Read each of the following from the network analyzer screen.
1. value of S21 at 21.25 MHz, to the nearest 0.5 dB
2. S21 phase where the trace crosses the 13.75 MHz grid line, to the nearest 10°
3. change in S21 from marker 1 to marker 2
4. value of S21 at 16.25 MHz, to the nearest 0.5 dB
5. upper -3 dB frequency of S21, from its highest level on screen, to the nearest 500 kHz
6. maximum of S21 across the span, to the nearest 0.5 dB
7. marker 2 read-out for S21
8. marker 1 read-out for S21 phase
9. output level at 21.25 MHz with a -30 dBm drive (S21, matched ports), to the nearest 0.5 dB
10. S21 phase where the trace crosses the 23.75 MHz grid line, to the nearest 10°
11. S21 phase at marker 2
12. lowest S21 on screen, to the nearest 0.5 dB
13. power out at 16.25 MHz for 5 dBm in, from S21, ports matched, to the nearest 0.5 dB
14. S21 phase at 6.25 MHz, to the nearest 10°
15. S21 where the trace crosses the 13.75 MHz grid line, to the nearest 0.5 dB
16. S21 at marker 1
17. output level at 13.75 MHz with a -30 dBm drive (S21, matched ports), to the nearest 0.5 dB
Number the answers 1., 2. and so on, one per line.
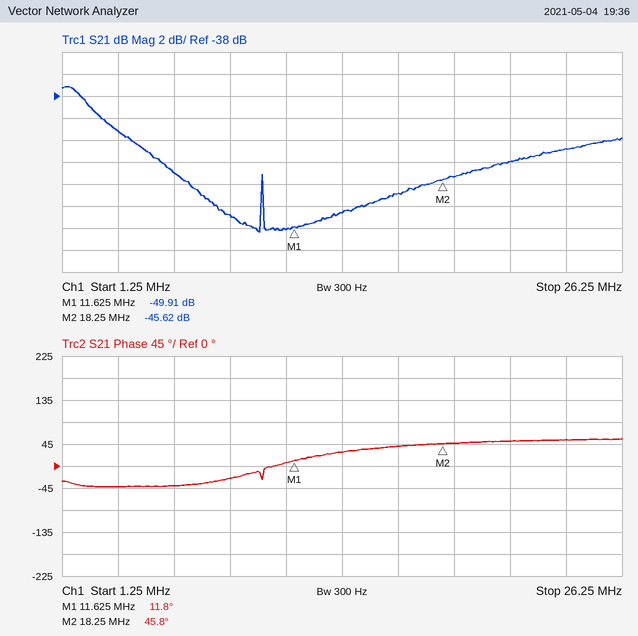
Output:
1. -44.0 dB
2. 30°
3. 4.29 dB
4. -47.0 dB
5. 3.0 MHz
6. -37.0 dB
7. -45.62 dB
8. 11.8°
9. -74.0 dBm
10. 50°
11. 45.8°
12. -50.5 dB
13. -42.0 dBm
14. -40°
15. -48.5 dB
16. -49.91 dB
17. -78.5 dBm
